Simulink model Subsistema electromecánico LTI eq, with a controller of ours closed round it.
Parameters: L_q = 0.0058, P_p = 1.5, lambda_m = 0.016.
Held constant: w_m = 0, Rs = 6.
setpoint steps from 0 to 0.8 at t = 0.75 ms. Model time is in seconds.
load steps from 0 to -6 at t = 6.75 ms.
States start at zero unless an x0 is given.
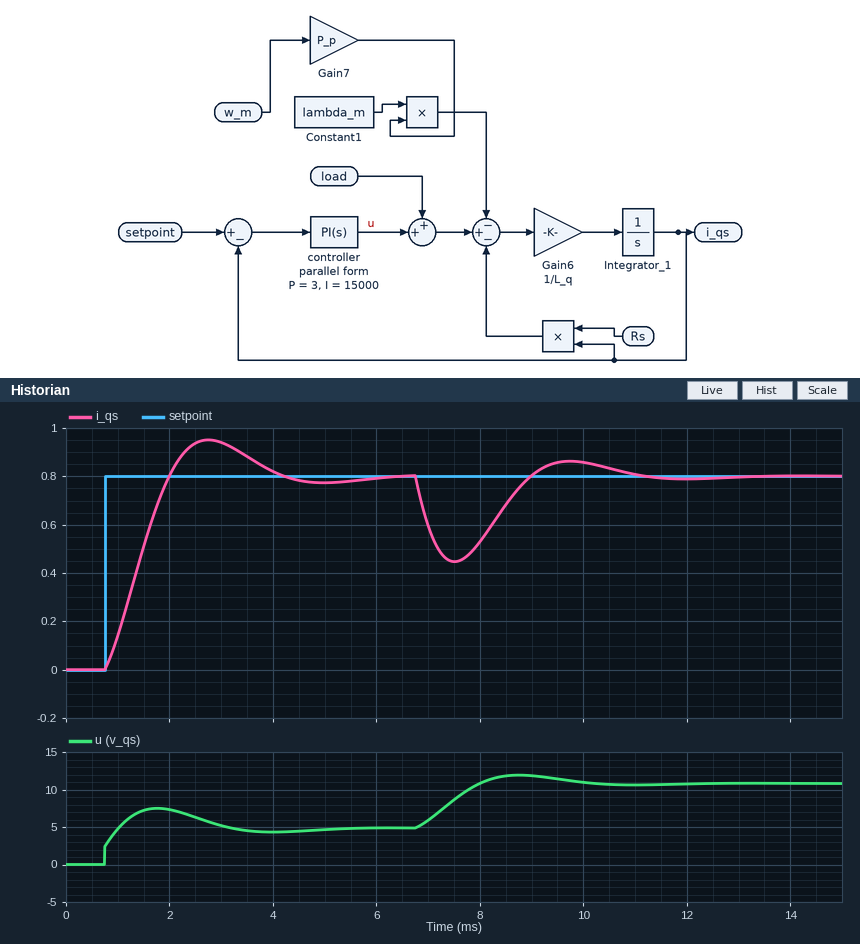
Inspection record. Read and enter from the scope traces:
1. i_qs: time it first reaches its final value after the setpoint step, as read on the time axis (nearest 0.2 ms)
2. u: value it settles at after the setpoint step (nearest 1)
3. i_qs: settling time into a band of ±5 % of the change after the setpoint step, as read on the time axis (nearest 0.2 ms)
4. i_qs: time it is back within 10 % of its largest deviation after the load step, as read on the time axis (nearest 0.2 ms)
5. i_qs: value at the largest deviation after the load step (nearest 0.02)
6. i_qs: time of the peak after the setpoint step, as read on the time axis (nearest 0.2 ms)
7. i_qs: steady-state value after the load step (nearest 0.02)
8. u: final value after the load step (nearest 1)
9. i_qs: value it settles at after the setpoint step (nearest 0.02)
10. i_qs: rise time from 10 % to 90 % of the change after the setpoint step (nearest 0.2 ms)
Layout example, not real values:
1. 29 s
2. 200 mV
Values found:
1. 2.0 ms
2. 5
3. 3.8 ms
4. 10.4 ms
5. 0.44
6. 2.8 ms
7. 0.80
8. 11
9. 0.80
10. 1.0 ms
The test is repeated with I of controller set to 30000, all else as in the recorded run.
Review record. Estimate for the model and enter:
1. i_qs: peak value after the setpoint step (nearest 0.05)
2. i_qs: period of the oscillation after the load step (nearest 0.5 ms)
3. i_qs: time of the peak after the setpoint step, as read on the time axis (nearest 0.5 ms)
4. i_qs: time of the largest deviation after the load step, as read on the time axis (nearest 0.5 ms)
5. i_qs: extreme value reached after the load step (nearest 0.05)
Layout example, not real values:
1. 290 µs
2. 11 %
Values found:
1. 1.05
2. 3.0 ms
3. 2.0 ms
4. 7.5 ms
5. 0.50
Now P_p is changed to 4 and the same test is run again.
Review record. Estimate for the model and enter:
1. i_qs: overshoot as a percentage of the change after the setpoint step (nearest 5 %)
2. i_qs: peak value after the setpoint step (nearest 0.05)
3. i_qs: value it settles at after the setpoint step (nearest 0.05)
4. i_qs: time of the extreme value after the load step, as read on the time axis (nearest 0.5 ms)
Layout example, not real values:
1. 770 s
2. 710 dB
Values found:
1. 20 %
2. 0.95
3. 0.80
4. 7.5 ms
